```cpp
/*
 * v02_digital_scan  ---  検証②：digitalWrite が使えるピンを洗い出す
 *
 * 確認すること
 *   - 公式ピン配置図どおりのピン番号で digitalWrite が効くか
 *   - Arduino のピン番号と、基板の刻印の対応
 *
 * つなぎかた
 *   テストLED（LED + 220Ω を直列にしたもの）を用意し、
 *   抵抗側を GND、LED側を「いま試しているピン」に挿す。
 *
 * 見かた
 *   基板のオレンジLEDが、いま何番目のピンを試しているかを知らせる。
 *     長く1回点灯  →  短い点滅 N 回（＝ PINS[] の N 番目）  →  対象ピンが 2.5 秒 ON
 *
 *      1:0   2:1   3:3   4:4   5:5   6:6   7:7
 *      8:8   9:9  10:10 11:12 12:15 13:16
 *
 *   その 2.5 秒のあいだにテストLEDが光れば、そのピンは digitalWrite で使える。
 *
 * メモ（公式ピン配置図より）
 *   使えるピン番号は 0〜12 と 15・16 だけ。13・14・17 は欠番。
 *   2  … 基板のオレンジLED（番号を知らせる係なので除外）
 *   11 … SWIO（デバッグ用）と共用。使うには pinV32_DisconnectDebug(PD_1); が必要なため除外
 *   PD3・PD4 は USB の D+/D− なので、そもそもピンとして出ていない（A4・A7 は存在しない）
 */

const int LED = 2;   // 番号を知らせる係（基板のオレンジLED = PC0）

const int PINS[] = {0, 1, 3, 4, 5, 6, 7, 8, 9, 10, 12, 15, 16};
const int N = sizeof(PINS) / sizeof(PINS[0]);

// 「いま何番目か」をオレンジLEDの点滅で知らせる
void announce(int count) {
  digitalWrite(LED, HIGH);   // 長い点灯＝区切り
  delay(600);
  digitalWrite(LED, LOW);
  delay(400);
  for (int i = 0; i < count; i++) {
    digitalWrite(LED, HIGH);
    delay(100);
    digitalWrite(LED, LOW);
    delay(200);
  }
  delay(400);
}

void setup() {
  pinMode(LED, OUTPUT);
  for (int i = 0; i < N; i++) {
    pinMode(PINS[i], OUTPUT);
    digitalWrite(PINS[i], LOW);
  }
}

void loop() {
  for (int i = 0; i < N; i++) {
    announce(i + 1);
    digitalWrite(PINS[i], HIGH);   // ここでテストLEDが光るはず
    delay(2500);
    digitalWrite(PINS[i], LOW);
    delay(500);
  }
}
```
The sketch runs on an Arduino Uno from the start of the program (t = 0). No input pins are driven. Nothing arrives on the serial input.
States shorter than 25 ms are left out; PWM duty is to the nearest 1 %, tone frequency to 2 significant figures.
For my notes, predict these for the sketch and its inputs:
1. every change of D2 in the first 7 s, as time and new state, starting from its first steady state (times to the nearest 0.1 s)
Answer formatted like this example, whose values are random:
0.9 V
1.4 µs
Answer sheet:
0 s high; 0.6 s low; 1 s high; 1.1 s low; 4.7 s high; 5.3 s low; 5.7 s high; 5.8 s low; 6 s high; 6.1 s low
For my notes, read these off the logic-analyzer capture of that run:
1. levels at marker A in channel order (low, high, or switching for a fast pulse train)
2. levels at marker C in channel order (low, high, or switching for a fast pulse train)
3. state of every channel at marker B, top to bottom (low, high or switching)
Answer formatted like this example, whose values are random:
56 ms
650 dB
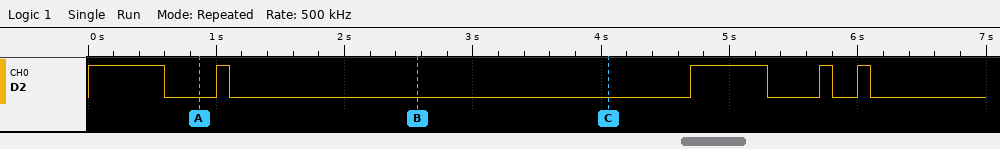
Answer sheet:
D2 low
D2 low
D2 low
